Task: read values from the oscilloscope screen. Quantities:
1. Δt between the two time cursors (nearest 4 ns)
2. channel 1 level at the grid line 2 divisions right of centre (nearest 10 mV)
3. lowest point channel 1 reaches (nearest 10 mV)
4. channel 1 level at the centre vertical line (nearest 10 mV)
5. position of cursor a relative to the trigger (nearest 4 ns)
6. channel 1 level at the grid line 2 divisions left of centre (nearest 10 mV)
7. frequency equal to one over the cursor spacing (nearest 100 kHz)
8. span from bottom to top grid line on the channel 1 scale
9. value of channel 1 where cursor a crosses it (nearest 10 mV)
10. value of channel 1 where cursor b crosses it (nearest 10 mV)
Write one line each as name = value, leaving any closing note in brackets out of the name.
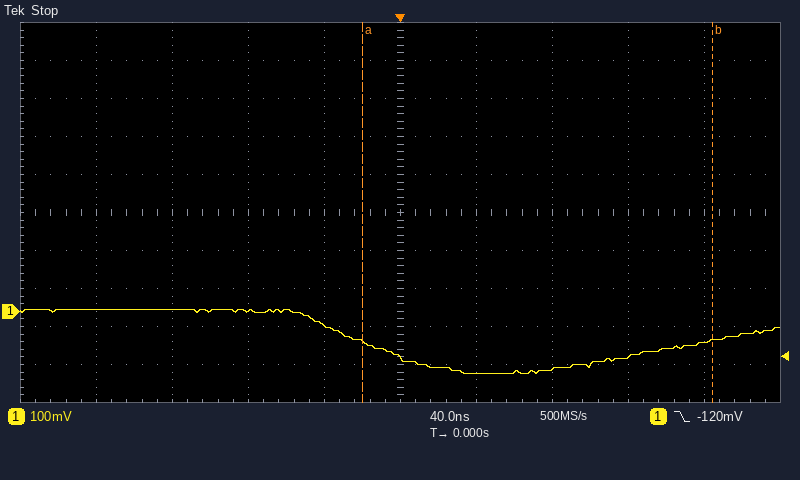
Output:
Δt between the two time cursors = 184 ns
channel 1 level at the grid line 2 divisions right of centre = -150 mV
lowest point channel 1 reaches = -160 mV
channel 1 level at the centre vertical line = -120 mV
position of cursor a relative to the trigger = -20 ns
channel 1 level at the grid line 2 divisions left of centre = 0 mV
frequency equal to one over the cursor spacing = 5.4 MHz
span from bottom to top grid line on the channel 1 scale = 1 V
value of channel 1 where cursor a crosses it = -80 mV
value of channel 1 where cursor b crosses it = -80 mV
